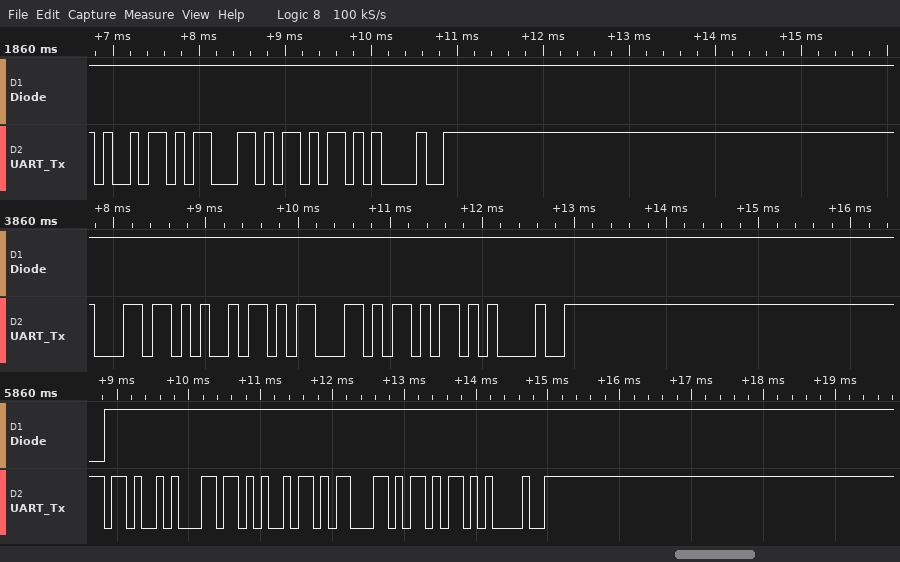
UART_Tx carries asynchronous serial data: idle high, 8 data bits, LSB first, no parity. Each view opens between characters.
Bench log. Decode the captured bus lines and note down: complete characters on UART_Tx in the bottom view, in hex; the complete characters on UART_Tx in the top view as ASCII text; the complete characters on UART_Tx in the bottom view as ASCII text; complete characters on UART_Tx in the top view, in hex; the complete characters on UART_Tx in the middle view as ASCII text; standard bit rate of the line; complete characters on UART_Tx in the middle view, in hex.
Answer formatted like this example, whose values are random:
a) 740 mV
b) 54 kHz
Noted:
a) 4B, 6C, 69, 63, 6B, 21
b) "ick!"
c) "Klick!"
d) 69, 63, 6B, 21
e) "lick!"
f) 9600 baud
g) 6C, 69, 63, 6B, 21
